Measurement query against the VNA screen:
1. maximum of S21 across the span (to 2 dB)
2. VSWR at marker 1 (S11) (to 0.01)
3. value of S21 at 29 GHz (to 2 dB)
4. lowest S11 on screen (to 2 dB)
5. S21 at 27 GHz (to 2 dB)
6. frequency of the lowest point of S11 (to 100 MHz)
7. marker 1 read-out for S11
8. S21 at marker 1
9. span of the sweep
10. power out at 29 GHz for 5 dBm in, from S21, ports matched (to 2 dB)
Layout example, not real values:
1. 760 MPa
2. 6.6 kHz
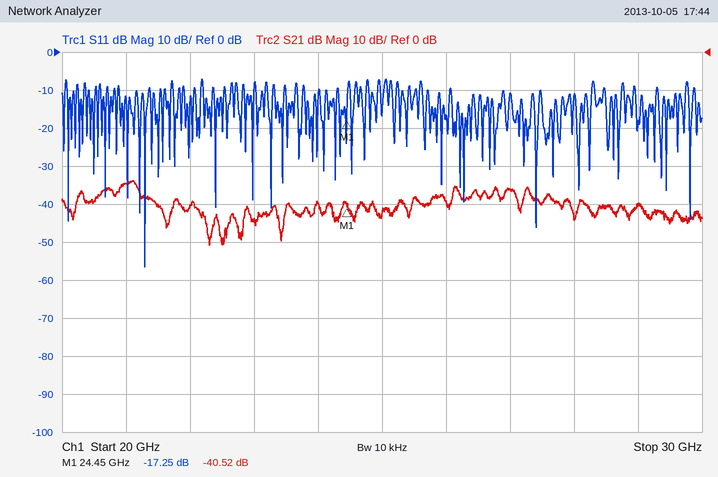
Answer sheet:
1. -34 dB
2. 1.32
3. -40 dB
4. -56 dB
5. -36 dB
6. 21.3 GHz
7. -17.25 dB
8. -40.52 dB
9. 10 GHz
10. -36 dBm
